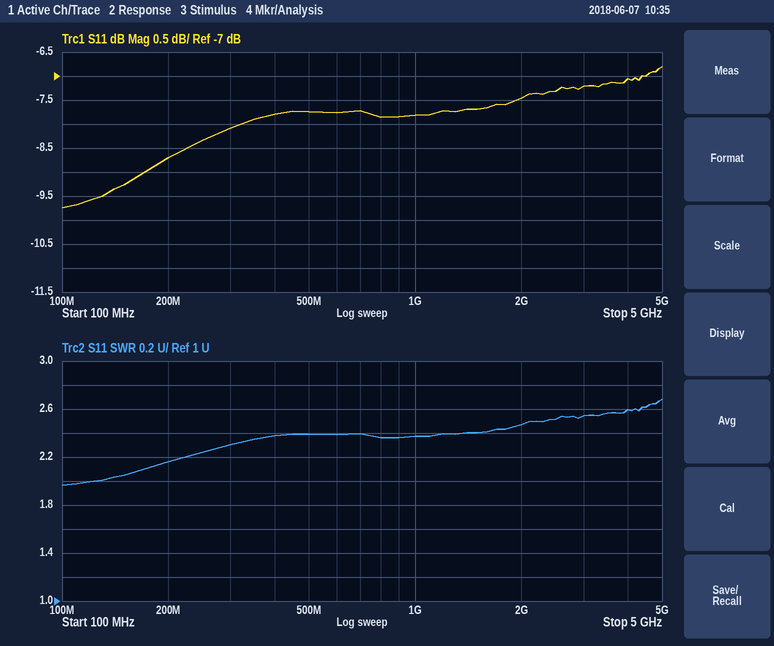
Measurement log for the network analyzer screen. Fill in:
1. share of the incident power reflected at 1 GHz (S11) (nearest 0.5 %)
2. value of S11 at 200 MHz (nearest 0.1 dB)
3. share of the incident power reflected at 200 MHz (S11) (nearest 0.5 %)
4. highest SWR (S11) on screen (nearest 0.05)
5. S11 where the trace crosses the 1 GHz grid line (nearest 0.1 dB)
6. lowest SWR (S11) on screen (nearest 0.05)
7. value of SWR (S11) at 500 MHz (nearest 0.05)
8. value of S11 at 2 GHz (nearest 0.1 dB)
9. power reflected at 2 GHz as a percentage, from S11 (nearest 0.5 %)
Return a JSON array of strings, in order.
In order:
["16.5 %", "-8.7 dB", "13.5 %", "2.70", "-7.8 dB", "1.95", "2.40", "-7.5 dB", "18.0 %"]
